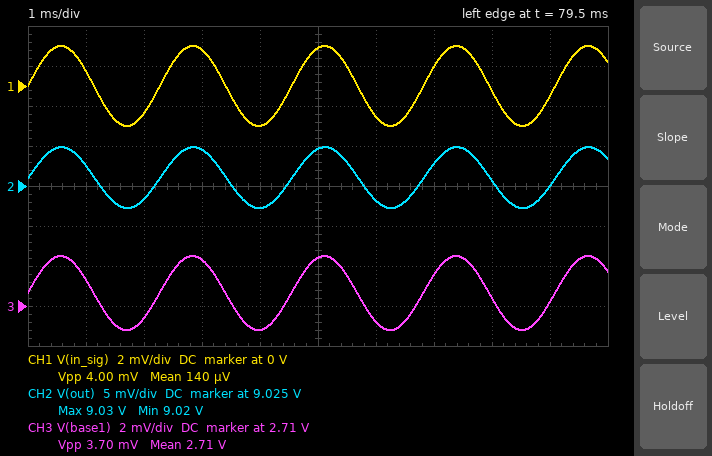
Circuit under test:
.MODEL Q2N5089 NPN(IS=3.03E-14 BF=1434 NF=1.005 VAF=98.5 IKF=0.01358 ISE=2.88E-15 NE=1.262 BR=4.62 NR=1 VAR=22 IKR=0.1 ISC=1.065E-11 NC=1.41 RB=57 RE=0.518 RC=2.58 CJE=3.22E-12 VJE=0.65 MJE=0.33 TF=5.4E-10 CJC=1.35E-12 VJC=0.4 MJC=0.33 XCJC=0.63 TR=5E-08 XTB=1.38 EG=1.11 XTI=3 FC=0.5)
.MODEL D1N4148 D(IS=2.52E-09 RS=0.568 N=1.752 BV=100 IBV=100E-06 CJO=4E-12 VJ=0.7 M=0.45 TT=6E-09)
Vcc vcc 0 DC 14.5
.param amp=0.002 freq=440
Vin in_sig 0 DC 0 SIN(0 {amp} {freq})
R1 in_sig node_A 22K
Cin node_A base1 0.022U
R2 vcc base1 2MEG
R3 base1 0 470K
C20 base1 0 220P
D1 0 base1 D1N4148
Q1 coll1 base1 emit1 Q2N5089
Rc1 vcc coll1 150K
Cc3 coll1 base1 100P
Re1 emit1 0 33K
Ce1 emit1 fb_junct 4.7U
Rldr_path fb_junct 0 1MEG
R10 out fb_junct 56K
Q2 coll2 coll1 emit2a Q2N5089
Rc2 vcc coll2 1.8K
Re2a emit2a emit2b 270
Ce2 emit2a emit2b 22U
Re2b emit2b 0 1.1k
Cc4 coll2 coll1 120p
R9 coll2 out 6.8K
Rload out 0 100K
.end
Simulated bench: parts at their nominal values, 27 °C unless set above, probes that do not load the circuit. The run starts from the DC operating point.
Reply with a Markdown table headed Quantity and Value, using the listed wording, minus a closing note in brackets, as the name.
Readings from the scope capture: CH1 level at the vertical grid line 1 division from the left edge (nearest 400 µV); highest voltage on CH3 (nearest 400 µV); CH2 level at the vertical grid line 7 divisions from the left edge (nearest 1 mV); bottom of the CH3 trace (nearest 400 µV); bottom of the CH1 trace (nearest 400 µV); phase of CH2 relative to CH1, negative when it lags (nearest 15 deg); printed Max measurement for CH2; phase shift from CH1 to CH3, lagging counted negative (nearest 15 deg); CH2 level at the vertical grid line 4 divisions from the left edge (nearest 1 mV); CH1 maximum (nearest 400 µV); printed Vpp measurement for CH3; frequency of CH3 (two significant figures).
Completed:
| Quantity | Value |
|---|---|
| CH1 level at the vertical grid line 1 division from the left edge | 800 µV |
| highest voltage on CH3 | 2.7124 V |
| CH2 level at the vertical grid line 7 divisions from the left edge | 9.028 V |
| bottom of the CH3 trace | 2.7088 V |
| bottom of the CH1 trace | -2.0 mV |
| phase of CH2 relative to CH1, negative when it lags | 0 deg |
| printed Max measurement for CH2 | 9.03 V |
| phase shift from CH1 to CH3, lagging counted negative | 0 deg |
| CH2 level at the vertical grid line 4 divisions from the left edge | 9.022 V |
| CH1 maximum | 2.0 mV |
| printed Vpp measurement for CH3 | 3.70 mV |
| frequency of CH3 | 440 Hz |
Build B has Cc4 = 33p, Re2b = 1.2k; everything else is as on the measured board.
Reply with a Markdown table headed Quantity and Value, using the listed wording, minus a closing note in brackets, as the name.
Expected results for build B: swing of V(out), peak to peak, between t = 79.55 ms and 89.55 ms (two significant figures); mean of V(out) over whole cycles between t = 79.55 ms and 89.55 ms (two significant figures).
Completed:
| Quantity | Value |
|---|---|
| swing of V(out), peak to peak, between t = 79.55 ms and 89.55 ms | 7.5 mV |
| mean of V(out) over whole cycles between t = 79.55 ms and 89.55 ms | 9.3 V |
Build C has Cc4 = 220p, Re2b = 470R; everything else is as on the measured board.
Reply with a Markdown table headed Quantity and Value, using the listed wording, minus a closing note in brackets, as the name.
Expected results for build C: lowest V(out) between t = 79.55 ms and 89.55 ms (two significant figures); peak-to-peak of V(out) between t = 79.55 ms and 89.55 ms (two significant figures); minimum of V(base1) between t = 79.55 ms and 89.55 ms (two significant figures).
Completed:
| Quantity | Value |
|---|---|
| lowest V(out) between t = 79.55 ms and 89.55 ms | 6.4 V |
| peak-to-peak of V(out) between t = 79.55 ms and 89.55 ms | 8.6 mV |
| minimum of V(base1) between t = 79.55 ms and 89.55 ms | 2.7 V |
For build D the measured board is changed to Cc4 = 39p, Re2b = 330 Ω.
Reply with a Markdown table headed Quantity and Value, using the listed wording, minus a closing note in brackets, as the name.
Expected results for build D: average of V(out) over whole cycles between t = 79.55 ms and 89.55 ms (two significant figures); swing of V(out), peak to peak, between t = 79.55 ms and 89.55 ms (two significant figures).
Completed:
| Quantity | Value |
|---|---|
| average of V(out) over whole cycles between t = 79.55 ms and 89.55 ms | 5.3 V |
| swing of V(out), peak to peak, between t = 79.55 ms and 89.55 ms | 8.8 mV |
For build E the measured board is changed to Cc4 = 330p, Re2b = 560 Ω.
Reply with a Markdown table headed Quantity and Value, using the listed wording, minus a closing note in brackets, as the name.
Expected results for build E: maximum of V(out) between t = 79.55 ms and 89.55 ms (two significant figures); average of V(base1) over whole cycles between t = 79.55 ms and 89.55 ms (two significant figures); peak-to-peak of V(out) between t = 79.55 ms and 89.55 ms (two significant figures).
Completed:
| Quantity | Value |
|---|---|
| maximum of V(out) between t = 79.55 ms and 89.55 ms | 6.9 V |
| average of V(base1) over whole cycles between t = 79.55 ms and 89.55 ms | 2.7 V |
| peak-to-peak of V(out) between t = 79.55 ms and 89.55 ms | 8.4 mV |
